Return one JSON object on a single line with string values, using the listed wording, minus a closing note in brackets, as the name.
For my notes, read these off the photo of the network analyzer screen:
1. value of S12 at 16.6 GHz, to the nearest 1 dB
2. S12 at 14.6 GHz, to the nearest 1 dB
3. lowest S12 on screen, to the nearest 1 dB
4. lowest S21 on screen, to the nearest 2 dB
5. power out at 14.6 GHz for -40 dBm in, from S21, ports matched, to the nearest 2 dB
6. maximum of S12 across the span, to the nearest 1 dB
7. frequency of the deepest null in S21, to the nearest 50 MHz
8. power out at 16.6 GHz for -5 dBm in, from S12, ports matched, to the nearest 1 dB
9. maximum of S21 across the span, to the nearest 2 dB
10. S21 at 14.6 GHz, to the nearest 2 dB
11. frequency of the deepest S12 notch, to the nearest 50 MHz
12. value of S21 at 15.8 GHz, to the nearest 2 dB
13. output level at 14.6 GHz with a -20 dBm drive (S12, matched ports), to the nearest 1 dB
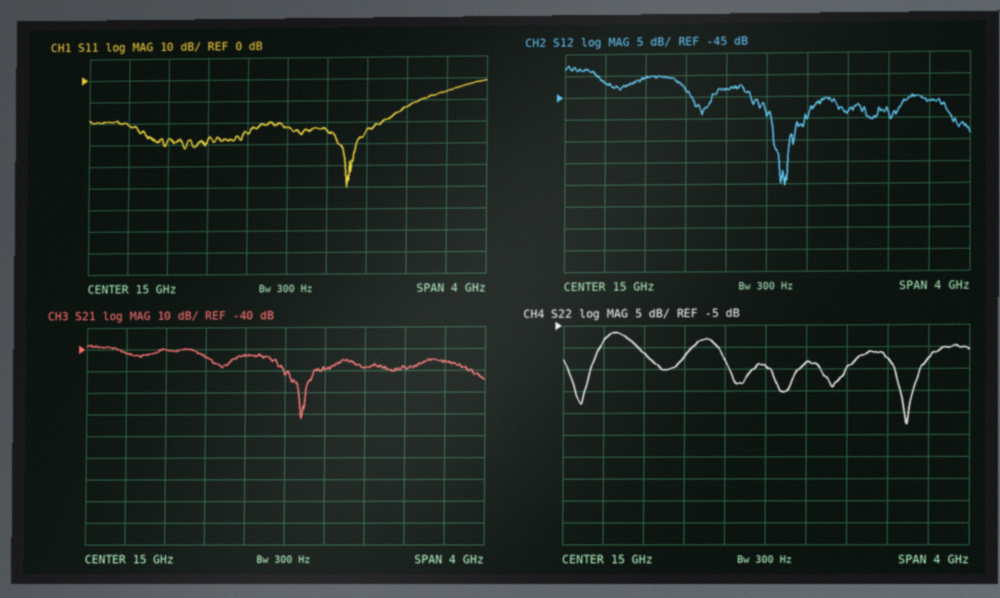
{"value of S12 at 16.6 GHz, to the nearest 1 dB": "-46 dB", "S12 at 14.6 GHz, to the nearest 1 dB": "-43 dB", "lowest S12 on screen, to the nearest 1 dB": "-65 dB", "lowest S21 on screen, to the nearest 2 dB": "-72 dB", "power out at 14.6 GHz for -40 dBm in, from S21, ports matched, to the nearest 2 dB": "-82 dBm", "maximum of S12 across the span, to the nearest 1 dB": "-38 dB", "frequency of the deepest null in S21, to the nearest 50 MHz": "15.15 GHz", "power out at 16.6 GHz for -5 dBm in, from S12, ports matched, to the nearest 1 dB": "-51 dBm", "maximum of S21 across the span, to the nearest 2 dB": "-38 dB", "S21 at 14.6 GHz, to the nearest 2 dB": "-42 dB", "frequency of the deepest S12 notch, to the nearest 50 MHz": "15.20 GHz", "value of S21 at 15.8 GHz, to the nearest 2 dB": "-48 dB", "output level at 14.6 GHz with a -20 dBm drive (S12, matched ports), to the nearest 1 dB": "-63 dBm"}
